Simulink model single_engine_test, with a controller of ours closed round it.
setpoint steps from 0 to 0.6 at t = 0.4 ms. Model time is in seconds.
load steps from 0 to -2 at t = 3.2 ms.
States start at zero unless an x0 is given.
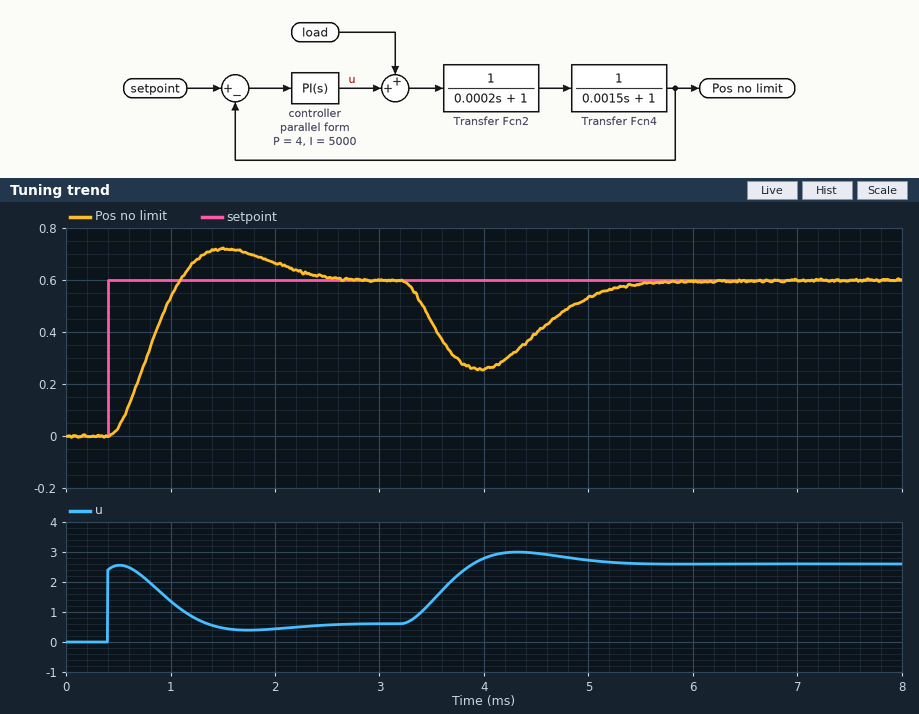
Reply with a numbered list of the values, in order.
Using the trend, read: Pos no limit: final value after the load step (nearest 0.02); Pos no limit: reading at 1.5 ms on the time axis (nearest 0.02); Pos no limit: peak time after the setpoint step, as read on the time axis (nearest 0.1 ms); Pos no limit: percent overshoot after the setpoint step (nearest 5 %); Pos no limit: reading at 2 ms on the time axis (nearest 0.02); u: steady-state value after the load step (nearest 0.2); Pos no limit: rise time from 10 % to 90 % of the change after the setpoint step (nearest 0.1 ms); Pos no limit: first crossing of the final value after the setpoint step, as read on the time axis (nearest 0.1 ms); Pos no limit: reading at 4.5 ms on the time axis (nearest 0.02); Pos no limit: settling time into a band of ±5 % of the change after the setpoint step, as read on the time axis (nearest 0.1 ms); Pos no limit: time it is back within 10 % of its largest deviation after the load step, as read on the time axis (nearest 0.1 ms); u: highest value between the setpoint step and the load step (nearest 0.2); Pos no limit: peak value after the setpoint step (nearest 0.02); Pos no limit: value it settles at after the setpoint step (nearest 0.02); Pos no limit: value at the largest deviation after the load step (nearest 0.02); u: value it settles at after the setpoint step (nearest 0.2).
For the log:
1. 0.60
2. 0.72
3. 1.5 ms
4. 20 %
5. 0.66
6. 2.6
7. 0.5 ms
8. 1.1 ms
9. 0.40
10. 2.3 ms
11. 5.2 ms
12. 2.6
13. 0.72
14. 0.60
15. 0.26
16. 0.6
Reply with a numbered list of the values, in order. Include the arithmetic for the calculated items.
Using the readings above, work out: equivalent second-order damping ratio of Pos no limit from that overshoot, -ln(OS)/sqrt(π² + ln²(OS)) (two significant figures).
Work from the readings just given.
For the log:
1. ln(0.2) = -1.609; 1.609 / sqrt(9.870 + 2.590) = 0.46
